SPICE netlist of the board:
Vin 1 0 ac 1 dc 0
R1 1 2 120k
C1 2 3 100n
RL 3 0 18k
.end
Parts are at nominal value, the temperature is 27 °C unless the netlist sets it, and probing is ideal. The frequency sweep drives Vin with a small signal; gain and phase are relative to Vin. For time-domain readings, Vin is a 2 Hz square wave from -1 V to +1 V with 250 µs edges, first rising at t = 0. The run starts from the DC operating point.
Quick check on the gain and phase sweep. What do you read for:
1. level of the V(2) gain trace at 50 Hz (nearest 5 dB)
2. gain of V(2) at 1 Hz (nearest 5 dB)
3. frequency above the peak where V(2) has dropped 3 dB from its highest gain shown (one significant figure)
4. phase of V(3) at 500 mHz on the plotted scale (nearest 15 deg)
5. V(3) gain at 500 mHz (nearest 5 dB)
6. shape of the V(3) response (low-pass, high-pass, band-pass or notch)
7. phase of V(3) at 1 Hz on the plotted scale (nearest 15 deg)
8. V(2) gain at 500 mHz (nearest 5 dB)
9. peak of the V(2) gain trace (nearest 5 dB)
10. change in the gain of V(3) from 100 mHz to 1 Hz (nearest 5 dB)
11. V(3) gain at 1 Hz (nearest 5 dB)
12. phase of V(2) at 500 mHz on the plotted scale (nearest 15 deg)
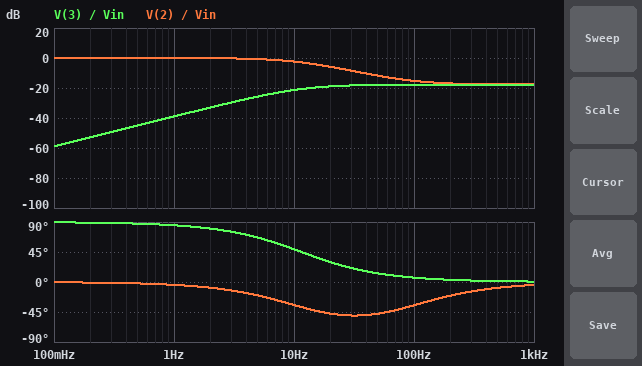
-10 dB
0 dB
10 Hz
90 deg
-45 dB
high-pass
90 deg
0 dB
0 dB
20 dB
-40 dB
0 deg
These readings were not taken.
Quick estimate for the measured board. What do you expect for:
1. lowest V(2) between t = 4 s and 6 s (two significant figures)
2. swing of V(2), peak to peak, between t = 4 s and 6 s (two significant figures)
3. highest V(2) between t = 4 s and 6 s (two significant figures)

-1.0 V
2.0 V
1.0 V
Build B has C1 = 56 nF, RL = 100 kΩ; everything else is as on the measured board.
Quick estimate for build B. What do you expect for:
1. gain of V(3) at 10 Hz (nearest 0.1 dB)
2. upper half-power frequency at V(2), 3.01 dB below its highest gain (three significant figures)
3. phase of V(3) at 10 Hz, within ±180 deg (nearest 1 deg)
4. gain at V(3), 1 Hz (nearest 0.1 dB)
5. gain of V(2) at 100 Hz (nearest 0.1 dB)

-11.1 dB
16.9 Hz
52 deg
-29.1 dB
-6.6 dB
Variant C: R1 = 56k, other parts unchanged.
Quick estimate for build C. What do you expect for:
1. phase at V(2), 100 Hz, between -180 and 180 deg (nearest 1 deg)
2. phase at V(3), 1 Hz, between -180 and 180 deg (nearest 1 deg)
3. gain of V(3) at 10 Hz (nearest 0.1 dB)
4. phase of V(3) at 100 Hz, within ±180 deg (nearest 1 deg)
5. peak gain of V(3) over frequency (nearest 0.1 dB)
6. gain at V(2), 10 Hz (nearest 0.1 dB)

-29 deg
87 deg
-19.8 dB
12 deg
-12.3 dB
-0.8 dB
